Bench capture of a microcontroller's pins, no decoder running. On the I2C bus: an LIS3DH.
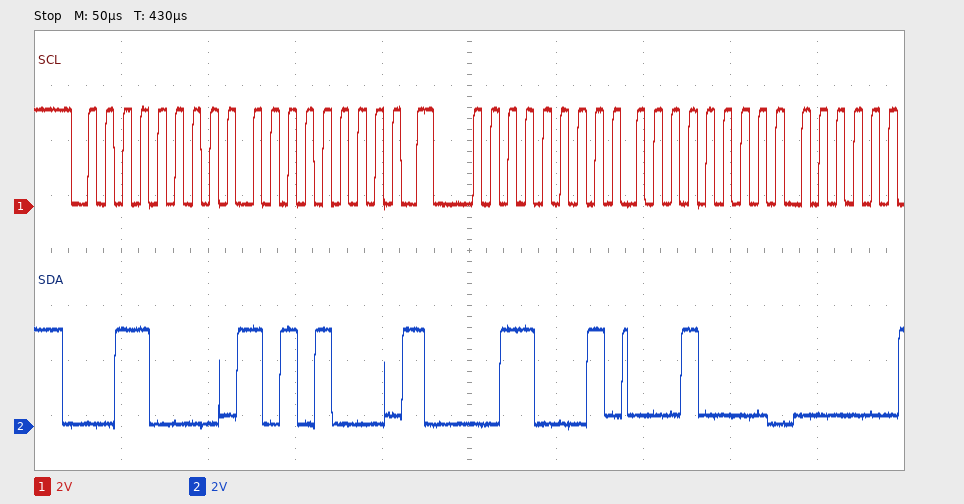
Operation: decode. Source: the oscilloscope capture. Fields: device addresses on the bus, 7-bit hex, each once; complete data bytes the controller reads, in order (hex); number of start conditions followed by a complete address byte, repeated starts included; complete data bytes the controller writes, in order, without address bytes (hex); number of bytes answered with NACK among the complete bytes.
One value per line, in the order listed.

0x18
10
2
A8
0
